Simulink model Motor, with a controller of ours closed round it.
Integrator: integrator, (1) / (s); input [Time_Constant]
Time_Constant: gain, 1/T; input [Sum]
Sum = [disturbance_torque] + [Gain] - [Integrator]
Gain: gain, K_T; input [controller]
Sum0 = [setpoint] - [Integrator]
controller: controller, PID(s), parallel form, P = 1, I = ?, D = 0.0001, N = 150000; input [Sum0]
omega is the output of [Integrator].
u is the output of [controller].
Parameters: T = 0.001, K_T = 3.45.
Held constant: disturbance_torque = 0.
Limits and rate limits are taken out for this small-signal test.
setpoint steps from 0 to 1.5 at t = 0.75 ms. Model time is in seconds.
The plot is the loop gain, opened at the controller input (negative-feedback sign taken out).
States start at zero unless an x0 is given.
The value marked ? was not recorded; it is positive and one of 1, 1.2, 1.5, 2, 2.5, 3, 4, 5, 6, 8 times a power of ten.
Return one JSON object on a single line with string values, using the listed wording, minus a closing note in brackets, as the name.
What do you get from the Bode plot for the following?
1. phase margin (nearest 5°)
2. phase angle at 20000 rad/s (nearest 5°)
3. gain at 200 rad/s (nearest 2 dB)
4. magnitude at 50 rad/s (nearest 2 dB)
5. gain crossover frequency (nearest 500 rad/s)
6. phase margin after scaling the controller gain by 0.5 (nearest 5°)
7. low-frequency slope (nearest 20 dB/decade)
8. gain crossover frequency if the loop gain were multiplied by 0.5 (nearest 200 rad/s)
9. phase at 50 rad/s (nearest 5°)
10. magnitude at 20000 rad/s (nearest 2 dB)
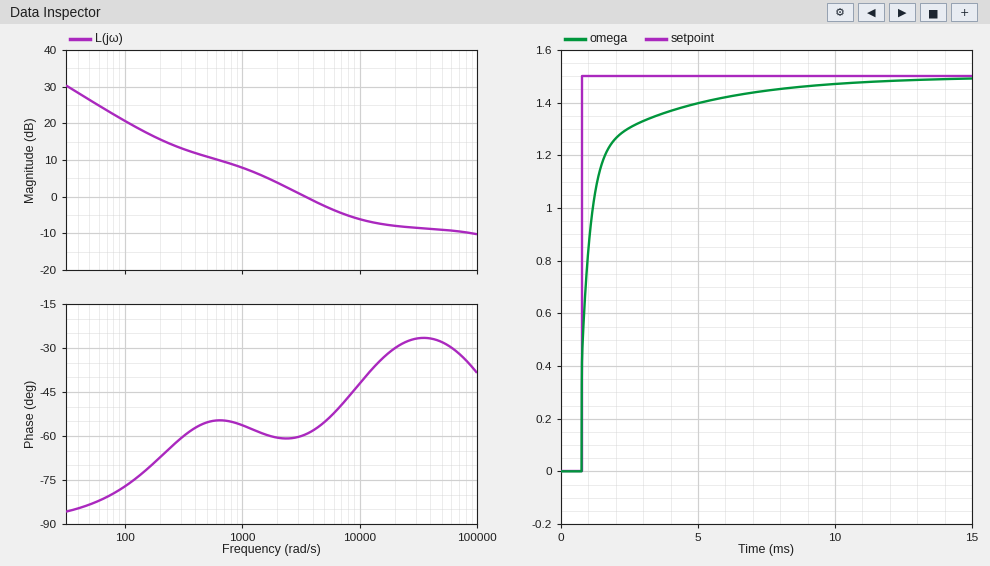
{"phase margin": "120°", "phase angle at 20000 rad/s": "-30°", "gain at 200 rad/s": "16 dB", "magnitude at 50 rad/s": "26 dB", "gain crossover frequency": "3500 rad/s", "phase margin after scaling the controller gain by 0.5": "120°", "low-frequency slope": "-20 dB/decade", "gain crossover frequency if the loop gain were multiplied by 0.5": "1400 rad/s", "phase at 50 rad/s": "-85°", "magnitude at 20000 rad/s": "-8 dB"}
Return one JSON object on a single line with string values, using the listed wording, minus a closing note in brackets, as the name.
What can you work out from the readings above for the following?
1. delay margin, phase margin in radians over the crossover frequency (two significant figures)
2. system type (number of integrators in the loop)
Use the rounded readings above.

{"delay margin, phase margin in radians over the crossover frequency": "0.00060 s", "system type": "1"}
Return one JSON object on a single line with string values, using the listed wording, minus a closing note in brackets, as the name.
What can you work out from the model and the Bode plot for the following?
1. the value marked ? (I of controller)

{"the value marked ?": "300"}
